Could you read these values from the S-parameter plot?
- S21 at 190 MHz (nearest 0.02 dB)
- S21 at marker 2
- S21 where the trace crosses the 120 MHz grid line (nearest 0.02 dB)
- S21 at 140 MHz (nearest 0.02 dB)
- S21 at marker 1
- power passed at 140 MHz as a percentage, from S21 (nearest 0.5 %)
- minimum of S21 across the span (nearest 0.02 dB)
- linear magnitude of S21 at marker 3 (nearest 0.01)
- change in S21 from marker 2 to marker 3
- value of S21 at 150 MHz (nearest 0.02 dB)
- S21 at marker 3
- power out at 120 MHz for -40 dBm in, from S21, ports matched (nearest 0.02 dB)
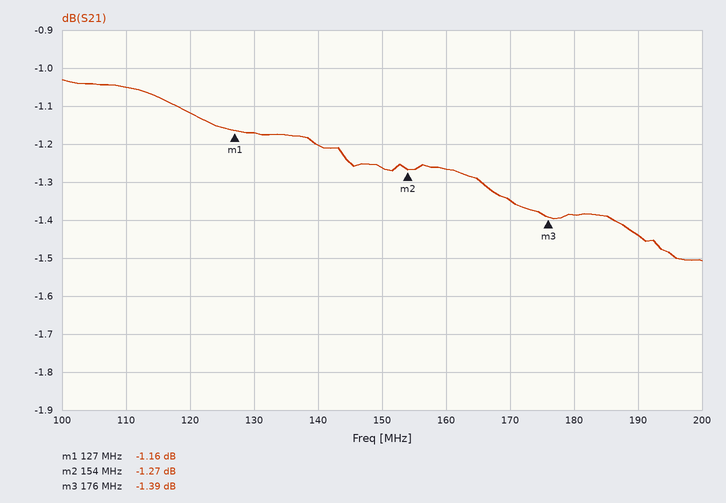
-1.44 dB
-1.27 dB
-1.12 dB
-1.20 dB
-1.16 dB
76.0 %
-1.50 dB
0.85
-0.12 dB
-1.26 dB
-1.39 dB
-41.12 dBm
